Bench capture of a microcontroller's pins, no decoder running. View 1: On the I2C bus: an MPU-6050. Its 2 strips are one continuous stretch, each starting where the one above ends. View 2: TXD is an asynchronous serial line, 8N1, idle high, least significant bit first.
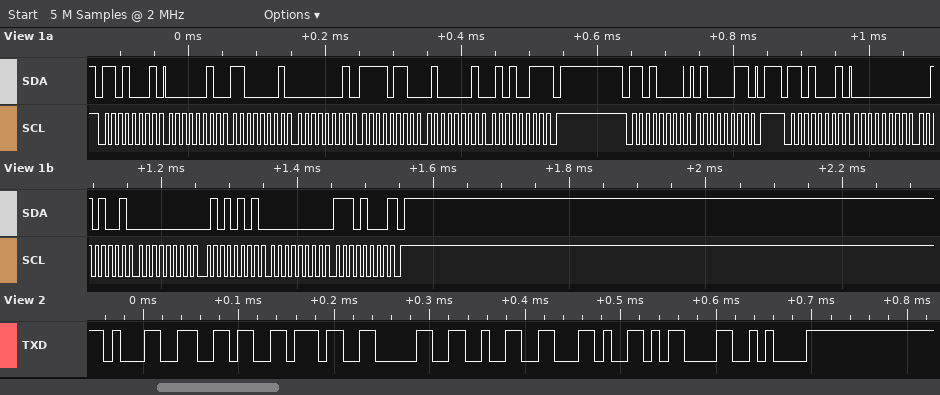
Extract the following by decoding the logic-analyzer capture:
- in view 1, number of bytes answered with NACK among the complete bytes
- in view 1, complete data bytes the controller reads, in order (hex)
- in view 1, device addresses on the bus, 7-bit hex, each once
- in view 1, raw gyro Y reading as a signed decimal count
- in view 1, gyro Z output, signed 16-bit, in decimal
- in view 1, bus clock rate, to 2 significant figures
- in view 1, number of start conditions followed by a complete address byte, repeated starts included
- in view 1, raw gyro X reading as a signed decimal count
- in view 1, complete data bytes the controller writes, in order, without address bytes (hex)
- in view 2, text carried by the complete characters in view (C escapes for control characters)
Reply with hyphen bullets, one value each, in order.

- 2
- 02 C1 01 F6 41 53 00 29 00 55 00 E8
- 0x68
- 85
- 232
- 100 kHz
- 3
- 41
- 43
- "16702,\r\n"
